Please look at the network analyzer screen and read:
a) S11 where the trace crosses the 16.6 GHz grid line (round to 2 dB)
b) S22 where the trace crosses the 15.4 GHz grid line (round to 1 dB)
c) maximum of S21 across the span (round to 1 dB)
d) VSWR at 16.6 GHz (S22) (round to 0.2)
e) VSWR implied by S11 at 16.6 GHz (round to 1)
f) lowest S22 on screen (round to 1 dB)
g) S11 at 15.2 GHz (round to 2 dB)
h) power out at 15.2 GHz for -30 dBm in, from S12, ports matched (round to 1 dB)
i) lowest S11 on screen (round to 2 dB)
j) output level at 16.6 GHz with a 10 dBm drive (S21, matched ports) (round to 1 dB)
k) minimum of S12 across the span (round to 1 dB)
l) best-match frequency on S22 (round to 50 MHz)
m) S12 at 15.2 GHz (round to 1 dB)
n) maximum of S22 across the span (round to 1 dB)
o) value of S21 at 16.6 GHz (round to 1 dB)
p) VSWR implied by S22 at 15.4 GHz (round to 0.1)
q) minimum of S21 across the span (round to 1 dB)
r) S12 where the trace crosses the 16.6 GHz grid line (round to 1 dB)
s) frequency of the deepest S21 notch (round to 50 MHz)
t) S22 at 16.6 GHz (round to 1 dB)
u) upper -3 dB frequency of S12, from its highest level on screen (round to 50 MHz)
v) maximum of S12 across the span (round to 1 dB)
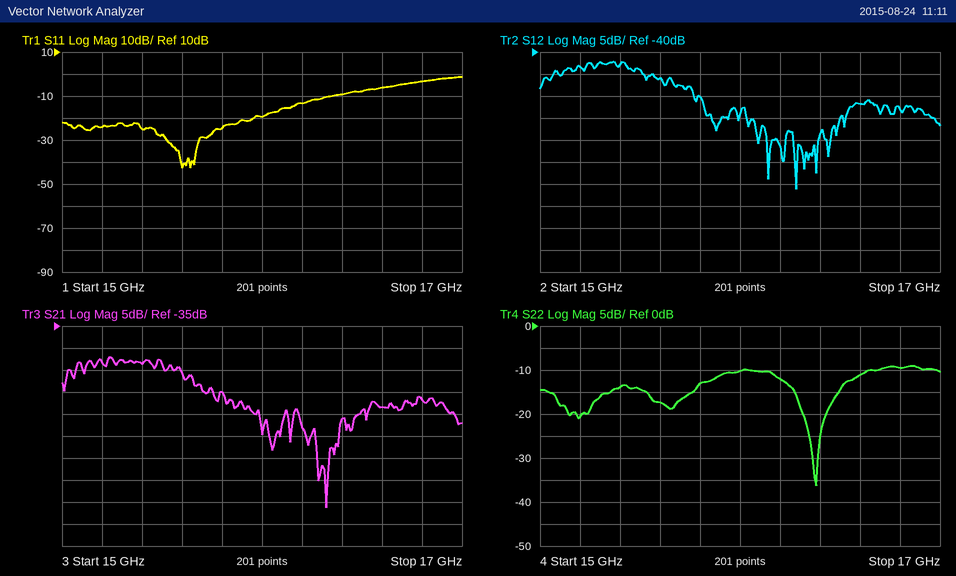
-6 dB
-14 dB
-42 dB
1.8
3
-36 dB
-24 dB
-73 dBm
-42 dB
-43 dBm
-71 dB
16.40 GHz
-43 dB
-9 dB
-53 dB
1.5
-76 dB
-52 dB
16.30 GHz
-11 dB
15.50 GHz
-42 dB
